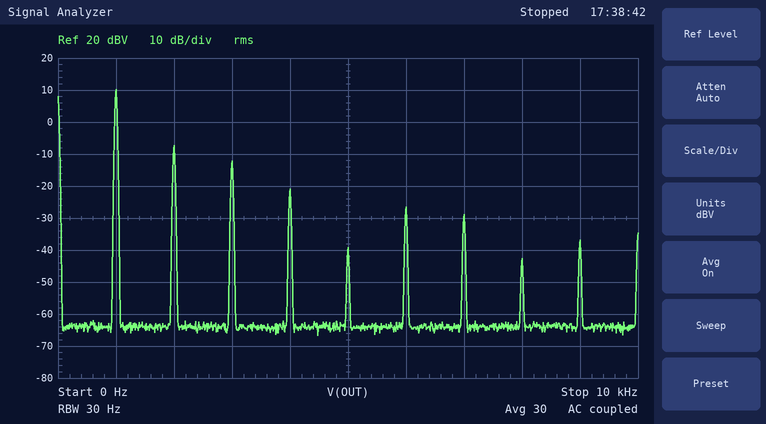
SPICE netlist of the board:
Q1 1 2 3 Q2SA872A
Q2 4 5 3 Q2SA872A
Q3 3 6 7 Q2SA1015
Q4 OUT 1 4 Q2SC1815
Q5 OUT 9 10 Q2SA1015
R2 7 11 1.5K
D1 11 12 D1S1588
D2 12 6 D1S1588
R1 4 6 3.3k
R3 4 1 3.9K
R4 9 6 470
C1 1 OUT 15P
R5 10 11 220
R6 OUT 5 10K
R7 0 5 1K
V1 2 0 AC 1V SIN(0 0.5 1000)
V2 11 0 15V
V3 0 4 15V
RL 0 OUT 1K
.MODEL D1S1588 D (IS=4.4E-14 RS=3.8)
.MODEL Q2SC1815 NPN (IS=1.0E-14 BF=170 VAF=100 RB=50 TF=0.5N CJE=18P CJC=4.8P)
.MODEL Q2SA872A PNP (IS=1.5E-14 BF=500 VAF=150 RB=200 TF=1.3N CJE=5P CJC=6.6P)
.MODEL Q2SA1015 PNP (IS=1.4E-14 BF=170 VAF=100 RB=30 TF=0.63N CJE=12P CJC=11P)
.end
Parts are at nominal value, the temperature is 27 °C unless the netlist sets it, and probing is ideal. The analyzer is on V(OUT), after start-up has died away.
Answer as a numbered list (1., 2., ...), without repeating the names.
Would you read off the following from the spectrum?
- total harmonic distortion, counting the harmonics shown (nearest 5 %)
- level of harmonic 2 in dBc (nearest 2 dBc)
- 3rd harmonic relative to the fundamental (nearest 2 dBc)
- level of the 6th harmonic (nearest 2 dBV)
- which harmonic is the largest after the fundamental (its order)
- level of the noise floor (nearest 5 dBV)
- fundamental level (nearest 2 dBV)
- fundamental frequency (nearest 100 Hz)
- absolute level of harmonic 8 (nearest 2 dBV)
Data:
1. 15 %
2. -18 dBc
3. -22 dBc
4. -26 dBV
5. 2
6. -65 dBV
7. 10 dBV
8. 1.0 kHz
9. -42 dBV
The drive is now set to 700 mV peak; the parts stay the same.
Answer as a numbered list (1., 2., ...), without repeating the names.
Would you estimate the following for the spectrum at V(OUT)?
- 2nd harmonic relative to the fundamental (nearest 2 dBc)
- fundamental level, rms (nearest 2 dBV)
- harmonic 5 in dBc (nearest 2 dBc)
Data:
1. -14 dBc
2. 12 dBV
3. -32 dBc
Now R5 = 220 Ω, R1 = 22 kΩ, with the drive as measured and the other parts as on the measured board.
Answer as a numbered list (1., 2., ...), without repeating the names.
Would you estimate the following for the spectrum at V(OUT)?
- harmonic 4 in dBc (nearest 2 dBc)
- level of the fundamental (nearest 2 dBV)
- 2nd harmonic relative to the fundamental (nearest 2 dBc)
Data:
1. -40 dBc
2. 10 dBV
3. -14 dBc
